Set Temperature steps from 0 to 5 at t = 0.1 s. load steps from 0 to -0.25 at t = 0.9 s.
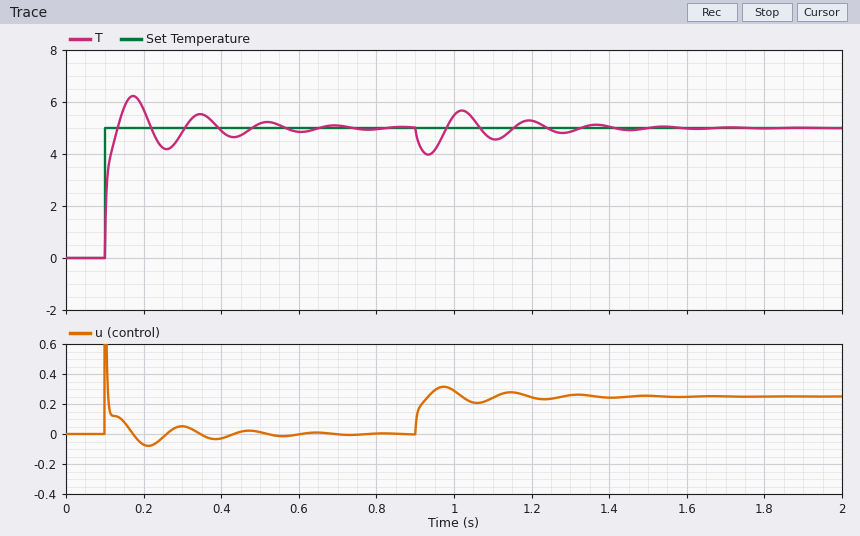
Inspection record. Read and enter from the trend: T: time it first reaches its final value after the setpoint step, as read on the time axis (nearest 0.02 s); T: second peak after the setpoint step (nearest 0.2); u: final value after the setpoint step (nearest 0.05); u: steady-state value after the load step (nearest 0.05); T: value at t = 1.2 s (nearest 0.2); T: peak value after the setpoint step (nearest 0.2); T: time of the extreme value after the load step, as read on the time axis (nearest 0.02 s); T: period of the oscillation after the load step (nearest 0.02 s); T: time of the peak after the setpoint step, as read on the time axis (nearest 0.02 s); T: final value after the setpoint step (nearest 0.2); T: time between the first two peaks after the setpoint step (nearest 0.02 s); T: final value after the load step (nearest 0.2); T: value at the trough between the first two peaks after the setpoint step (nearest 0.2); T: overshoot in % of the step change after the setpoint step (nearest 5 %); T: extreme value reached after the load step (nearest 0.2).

0.14 s
5.6
0.00
0.25
5.2
6.2
0.94 s
0.18 s
0.18 s
5.0
0.18 s
5.0
4.2
25 %
4.0
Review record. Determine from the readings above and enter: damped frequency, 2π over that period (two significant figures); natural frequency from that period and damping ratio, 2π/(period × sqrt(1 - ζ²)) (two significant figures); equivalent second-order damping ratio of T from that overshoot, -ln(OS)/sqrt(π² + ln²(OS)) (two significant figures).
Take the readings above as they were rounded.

35 rad/s
38 rad/s
0.40
